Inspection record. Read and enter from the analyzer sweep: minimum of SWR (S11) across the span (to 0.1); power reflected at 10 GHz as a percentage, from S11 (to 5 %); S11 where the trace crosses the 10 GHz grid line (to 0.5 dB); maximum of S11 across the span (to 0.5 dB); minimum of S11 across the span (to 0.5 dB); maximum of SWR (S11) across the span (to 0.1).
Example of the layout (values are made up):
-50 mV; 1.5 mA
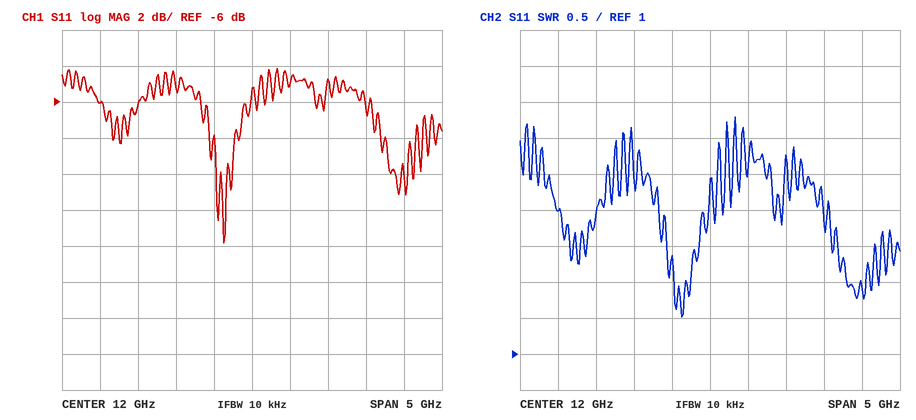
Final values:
1.5; 25 %; -6.0 dB; -4.0 dB; -14.0 dB; 4.3
